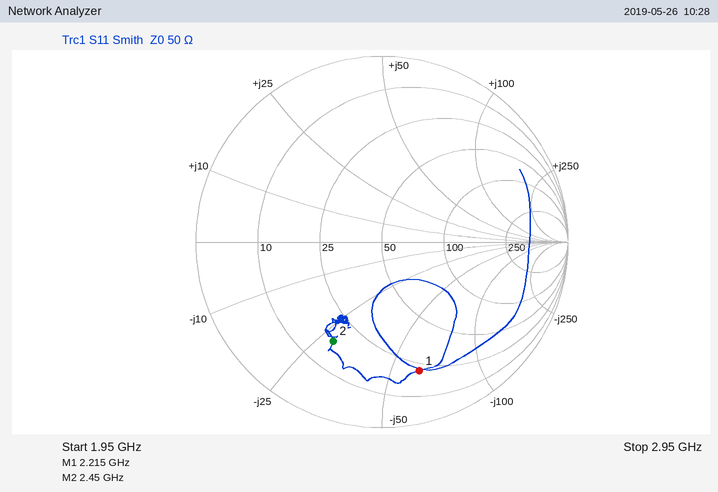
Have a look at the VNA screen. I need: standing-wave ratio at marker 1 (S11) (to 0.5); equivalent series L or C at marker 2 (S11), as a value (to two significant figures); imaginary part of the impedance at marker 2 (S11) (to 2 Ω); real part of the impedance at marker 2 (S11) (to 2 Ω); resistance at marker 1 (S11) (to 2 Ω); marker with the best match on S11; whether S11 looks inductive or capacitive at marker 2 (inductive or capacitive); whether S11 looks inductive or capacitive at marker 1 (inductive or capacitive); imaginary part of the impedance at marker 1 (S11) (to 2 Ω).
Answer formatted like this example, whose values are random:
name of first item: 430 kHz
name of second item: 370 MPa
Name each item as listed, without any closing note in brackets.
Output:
standing-wave ratio at marker 1 (S11): 6.0
equivalent series L or C at marker 2 (S11), as a value: 2.3 pF
imaginary part of the impedance at marker 2 (S11): -28 Ω
real part of the impedance at marker 2 (S11): 18 Ω
resistance at marker 1 (S11): 22 Ω
marker with the best match on S11: marker 2
whether S11 looks inductive or capacitive at marker 2: capacitive
whether S11 looks inductive or capacitive at marker 1: capacitive
imaginary part of the impedance at marker 1 (S11): -62 Ω
